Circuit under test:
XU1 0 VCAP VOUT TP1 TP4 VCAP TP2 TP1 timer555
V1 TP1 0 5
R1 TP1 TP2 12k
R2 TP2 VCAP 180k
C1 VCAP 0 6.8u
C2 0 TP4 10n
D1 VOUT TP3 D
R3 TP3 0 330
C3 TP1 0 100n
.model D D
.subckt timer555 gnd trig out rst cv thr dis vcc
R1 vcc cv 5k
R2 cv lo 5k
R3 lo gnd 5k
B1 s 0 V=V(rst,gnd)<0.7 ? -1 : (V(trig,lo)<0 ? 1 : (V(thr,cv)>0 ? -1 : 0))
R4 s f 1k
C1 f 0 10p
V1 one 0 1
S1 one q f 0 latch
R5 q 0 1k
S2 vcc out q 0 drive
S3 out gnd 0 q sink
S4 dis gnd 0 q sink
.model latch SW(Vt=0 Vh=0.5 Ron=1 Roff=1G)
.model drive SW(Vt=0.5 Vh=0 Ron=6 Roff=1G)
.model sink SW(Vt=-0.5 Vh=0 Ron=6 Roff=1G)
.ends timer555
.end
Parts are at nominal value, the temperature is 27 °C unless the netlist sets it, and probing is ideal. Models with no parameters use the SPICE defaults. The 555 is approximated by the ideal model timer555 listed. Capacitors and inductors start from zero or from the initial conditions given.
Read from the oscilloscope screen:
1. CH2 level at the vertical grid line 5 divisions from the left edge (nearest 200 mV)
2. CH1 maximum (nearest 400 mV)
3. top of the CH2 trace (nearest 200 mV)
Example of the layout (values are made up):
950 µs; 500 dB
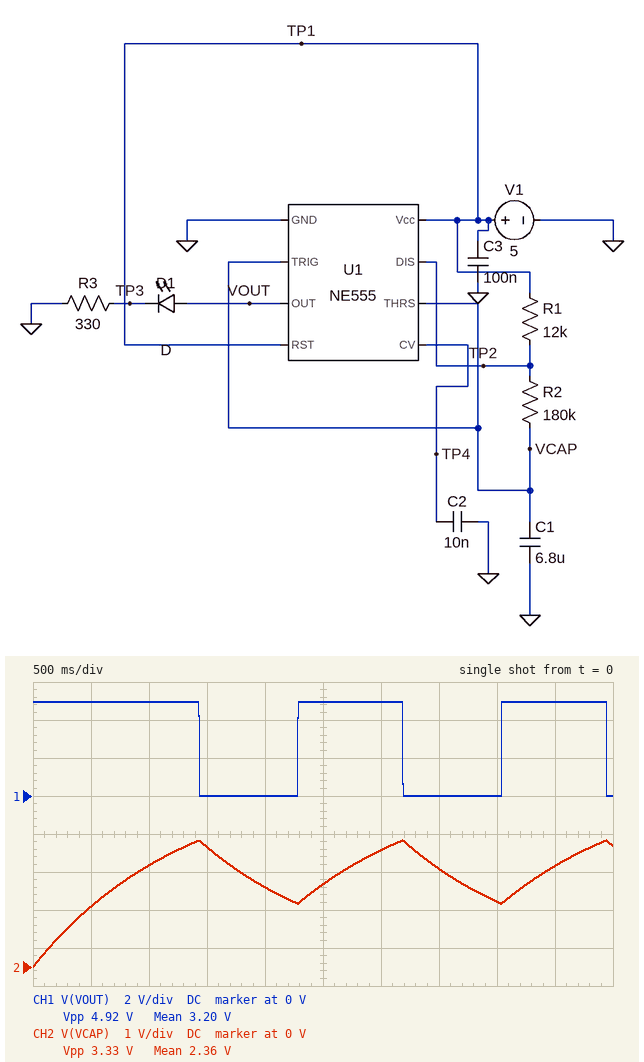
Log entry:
2.2 V; 4.8 V; 3.4 V
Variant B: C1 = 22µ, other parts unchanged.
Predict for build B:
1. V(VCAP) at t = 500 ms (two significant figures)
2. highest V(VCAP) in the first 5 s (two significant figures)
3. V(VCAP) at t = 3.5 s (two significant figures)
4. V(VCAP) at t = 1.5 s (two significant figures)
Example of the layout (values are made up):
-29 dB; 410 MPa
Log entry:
560 mV; 3.3 V; 2.8 V; 1.5 V
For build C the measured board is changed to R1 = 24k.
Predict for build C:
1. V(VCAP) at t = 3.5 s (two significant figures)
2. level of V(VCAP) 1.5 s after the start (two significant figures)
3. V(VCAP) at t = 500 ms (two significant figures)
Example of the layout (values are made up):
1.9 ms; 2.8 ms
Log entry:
2.9 V; 3.3 V; 1.5 V
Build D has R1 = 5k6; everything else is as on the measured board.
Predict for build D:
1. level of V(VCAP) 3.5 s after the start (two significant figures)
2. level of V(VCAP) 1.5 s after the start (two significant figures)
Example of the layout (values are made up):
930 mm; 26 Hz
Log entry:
2.4 V; 3.0 V
